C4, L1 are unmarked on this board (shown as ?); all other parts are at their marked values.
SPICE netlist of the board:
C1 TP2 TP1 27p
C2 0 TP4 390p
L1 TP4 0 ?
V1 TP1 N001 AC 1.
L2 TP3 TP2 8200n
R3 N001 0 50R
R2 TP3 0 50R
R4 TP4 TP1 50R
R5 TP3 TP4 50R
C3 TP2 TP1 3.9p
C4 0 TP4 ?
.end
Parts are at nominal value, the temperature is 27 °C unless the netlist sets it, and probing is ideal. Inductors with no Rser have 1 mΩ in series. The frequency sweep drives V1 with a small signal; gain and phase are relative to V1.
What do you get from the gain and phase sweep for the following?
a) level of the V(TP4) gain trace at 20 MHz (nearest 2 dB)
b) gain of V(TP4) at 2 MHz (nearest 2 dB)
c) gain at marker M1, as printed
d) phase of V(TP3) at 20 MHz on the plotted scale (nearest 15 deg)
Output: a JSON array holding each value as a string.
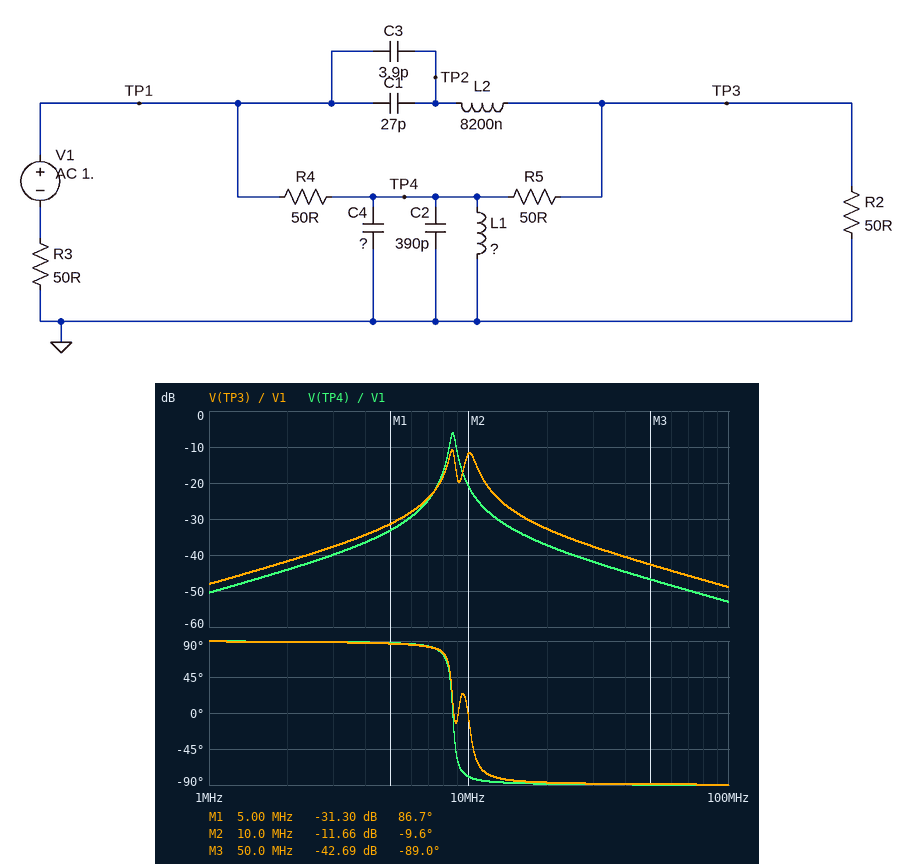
["-38 dB", "-44 dB", "-31.30 dB", "-90 deg"]
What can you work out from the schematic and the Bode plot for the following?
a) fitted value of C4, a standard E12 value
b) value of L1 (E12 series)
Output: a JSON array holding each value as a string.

["6.8 nF", "47 nH"]
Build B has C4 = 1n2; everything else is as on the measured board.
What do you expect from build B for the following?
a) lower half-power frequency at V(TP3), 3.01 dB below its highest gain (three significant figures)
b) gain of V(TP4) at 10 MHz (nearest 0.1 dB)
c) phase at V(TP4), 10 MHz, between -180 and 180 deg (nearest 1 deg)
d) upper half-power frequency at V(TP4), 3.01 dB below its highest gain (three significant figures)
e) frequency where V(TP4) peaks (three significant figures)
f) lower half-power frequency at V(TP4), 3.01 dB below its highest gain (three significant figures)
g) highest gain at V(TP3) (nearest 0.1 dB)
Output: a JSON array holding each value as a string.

["9.45 MHz", "-27.6 dB", "85 deg", "19.4 MHz", "18.4 MHz", "17.4 MHz", "-11.9 dB"]
